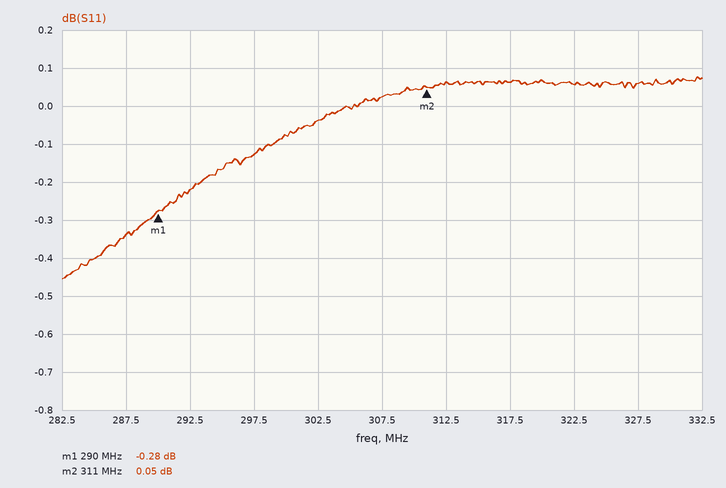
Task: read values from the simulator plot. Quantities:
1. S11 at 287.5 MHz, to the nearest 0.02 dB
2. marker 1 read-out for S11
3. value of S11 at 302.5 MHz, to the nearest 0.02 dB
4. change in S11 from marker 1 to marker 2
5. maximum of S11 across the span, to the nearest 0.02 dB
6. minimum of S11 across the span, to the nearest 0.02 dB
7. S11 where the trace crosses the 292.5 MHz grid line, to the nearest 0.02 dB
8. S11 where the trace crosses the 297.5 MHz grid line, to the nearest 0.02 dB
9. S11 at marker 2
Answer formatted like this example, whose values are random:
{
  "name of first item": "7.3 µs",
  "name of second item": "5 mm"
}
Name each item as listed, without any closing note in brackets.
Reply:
{
  "S11 at 287.5 MHz, to the nearest 0.02 dB": "-0.34 dB",
  "marker 1 read-out for S11": "-0.28 dB",
  "value of S11 at 302.5 MHz, to the nearest 0.02 dB": "-0.04 dB",
  "change in S11 from marker 1 to marker 2": "0.33 dB",
  "maximum of S11 across the span, to the nearest 0.02 dB": "0.08 dB",
  "minimum of S11 across the span, to the nearest 0.02 dB": "-0.46 dB",
  "S11 where the trace crosses the 292.5 MHz grid line, to the nearest 0.02 dB": "-0.22 dB",
  "S11 where the trace crosses the 297.5 MHz grid line, to the nearest 0.02 dB": "-0.12 dB",
  "S11 at marker 2": "0.05 dB"
}
